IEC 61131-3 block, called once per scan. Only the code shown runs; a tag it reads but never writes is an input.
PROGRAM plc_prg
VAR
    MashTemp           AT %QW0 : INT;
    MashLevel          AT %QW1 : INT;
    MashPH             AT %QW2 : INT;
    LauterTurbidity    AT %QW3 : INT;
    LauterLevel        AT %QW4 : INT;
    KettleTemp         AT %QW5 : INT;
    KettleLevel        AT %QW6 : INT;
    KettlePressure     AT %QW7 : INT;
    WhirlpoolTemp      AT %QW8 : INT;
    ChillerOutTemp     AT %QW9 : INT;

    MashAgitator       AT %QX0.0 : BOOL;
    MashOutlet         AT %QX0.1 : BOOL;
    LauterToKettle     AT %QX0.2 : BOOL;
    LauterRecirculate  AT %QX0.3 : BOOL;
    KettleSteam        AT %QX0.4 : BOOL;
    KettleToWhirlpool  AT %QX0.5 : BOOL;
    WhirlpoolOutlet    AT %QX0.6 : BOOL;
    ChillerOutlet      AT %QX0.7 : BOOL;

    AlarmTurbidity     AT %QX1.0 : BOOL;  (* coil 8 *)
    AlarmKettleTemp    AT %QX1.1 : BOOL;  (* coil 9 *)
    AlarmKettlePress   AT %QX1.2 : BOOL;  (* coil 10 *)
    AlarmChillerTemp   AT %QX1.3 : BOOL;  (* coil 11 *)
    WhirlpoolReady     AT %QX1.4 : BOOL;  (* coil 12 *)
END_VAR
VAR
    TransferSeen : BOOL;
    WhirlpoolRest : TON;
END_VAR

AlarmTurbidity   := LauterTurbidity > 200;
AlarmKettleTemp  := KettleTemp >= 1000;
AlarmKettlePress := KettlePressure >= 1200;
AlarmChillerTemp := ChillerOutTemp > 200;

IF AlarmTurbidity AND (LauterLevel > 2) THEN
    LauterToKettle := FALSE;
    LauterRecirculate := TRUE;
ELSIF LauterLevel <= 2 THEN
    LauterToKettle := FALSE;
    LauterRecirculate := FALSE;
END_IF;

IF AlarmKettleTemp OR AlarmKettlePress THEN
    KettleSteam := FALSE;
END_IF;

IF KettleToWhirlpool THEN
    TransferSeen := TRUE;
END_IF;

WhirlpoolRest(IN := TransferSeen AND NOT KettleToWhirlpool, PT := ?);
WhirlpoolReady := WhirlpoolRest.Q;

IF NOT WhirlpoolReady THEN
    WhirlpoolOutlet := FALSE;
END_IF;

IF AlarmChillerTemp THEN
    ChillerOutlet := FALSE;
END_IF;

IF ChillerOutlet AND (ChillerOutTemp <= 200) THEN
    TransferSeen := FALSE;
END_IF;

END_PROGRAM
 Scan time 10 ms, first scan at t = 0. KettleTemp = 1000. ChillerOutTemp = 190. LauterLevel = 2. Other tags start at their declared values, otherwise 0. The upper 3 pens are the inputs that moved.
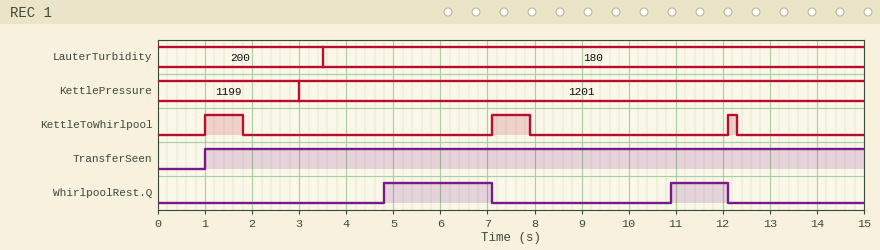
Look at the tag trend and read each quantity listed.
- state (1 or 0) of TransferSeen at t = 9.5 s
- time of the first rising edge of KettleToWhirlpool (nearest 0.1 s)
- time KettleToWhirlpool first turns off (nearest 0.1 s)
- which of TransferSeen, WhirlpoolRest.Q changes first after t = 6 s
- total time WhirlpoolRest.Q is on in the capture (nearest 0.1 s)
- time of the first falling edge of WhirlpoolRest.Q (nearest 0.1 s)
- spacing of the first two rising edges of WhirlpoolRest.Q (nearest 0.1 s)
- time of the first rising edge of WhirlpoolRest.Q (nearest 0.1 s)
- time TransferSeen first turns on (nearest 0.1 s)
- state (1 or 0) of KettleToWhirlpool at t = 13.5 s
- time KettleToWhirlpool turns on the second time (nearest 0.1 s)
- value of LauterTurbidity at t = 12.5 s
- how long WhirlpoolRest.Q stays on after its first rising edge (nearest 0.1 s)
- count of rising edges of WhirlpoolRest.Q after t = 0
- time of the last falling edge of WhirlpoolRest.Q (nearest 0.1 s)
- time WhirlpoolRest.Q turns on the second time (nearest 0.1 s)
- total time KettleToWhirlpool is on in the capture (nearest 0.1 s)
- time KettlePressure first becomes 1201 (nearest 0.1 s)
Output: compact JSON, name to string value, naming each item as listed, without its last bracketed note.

{"state (1 or 0) of TransferSeen at t = 9.5 s": "1", "time of the first rising edge of KettleToWhirlpool": "1.0 s", "time KettleToWhirlpool first turns off": "1.8 s", "which of TransferSeen, WhirlpoolRest.Q changes first after t = 6 s": "WhirlpoolRest.Q", "total time WhirlpoolRest.Q is on in the capture": "3.5 s", "time of the first falling edge of WhirlpoolRest.Q": "7.1 s", "spacing of the first two rising edges of WhirlpoolRest.Q": "6.1 s", "time of the first rising edge of WhirlpoolRest.Q": "4.8 s", "time TransferSeen first turns on": "1.0 s", "state (1 or 0) of KettleToWhirlpool at t = 13.5 s": "0", "time KettleToWhirlpool turns on the second time": "7.1 s", "value of LauterTurbidity at t = 12.5 s": "180", "how long WhirlpoolRest.Q stays on after its first rising edge": "2.3 s", "count of rising edges of WhirlpoolRest.Q after t = 0": "2", "time of the last falling edge of WhirlpoolRest.Q": "12.1 s", "time WhirlpoolRest.Q turns on the second time": "10.9 s", "total time KettleToWhirlpool is on in the capture": "1.8 s", "time KettlePressure first becomes 1201": "3.0 s"}
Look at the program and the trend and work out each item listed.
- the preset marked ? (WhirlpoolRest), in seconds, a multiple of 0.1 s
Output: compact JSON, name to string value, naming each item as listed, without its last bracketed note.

{"the preset marked ? (WhirlpoolRest), in seconds, a multiple of 0.1 s": "3.0 s"}
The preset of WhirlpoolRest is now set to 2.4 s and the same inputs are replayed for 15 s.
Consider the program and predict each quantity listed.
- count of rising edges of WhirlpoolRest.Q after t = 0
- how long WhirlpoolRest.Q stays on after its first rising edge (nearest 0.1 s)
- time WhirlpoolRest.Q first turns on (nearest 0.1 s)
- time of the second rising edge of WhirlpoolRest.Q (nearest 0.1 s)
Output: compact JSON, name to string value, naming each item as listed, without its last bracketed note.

{"count of rising edges of WhirlpoolRest.Q after t = 0": "3", "how long WhirlpoolRest.Q stays on after its first rising edge": "2.9 s", "time WhirlpoolRest.Q first turns on": "4.2 s", "time of the second rising edge of WhirlpoolRest.Q": "10.3 s"}
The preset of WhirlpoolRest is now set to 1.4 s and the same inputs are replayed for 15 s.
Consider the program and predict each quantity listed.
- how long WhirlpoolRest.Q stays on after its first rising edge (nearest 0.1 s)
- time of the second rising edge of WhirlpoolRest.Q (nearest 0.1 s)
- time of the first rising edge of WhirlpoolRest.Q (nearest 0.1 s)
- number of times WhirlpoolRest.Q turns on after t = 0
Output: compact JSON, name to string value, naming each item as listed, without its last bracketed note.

{"how long WhirlpoolRest.Q stays on after its first rising edge": "3.9 s", "time of the second rising edge of WhirlpoolRest.Q": "9.3 s", "time of the first rising edge of WhirlpoolRest.Q": "3.2 s", "number of times WhirlpoolRest.Q turns on after t = 0": "3"}
